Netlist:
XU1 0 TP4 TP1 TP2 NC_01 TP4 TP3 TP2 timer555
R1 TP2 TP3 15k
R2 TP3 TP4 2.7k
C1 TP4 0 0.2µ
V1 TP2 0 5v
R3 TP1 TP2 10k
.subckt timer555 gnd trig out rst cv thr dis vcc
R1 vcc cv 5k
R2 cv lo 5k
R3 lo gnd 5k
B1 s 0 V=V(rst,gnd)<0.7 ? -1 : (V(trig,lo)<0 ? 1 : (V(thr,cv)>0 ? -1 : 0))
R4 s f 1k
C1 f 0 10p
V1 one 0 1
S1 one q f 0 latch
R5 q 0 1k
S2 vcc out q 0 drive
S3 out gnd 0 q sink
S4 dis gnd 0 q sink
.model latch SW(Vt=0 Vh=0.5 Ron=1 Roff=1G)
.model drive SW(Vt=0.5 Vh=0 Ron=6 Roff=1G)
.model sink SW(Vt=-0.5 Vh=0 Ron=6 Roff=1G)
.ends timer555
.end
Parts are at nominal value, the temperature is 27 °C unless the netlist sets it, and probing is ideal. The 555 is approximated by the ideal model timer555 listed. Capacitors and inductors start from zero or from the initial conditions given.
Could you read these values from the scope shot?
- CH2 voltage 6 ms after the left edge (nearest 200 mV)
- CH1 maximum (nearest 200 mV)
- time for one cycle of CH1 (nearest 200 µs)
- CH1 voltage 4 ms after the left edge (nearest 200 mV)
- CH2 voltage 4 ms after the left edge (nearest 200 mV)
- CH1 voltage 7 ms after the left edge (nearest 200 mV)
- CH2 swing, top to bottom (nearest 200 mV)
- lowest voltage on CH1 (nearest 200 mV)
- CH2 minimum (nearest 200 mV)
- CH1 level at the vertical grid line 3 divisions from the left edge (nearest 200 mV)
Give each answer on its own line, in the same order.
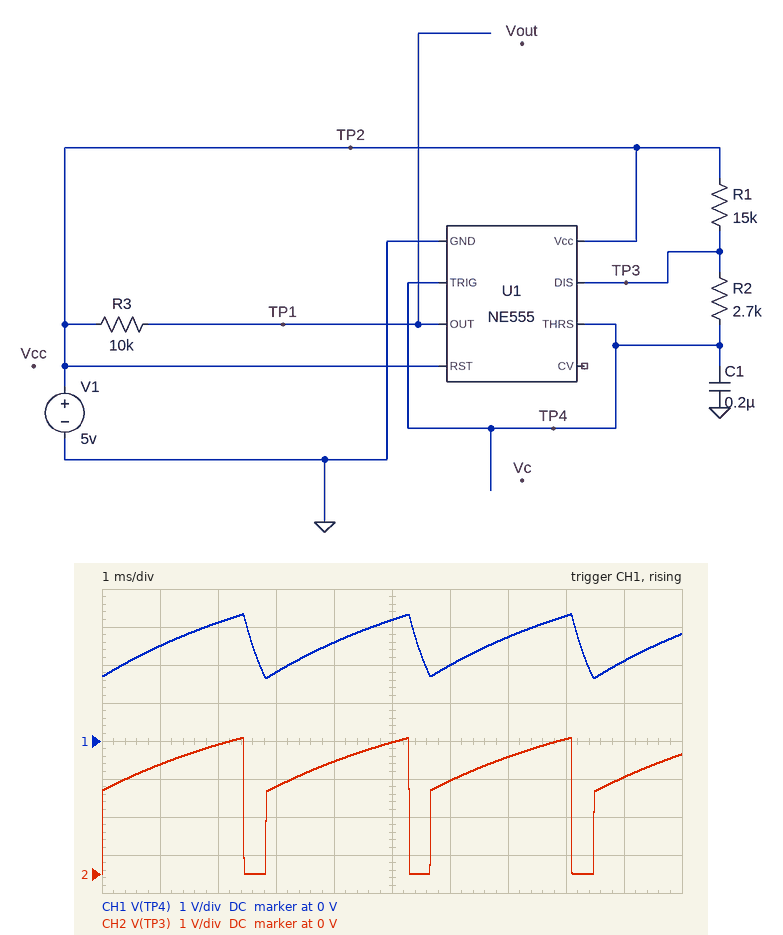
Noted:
2.4 V
3.4 V
2.8 ms
2.6 V
3.0 V
2.8 V
3.6 V
1.6 V
0 V
1.8 V
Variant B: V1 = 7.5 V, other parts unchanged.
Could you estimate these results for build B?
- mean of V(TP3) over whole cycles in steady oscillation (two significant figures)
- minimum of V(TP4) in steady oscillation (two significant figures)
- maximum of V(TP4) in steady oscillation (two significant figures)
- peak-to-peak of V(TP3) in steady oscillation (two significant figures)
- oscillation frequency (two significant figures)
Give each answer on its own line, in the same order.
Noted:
3.9 V
2.5 V
5.0 V
5.4 V
350 Hz
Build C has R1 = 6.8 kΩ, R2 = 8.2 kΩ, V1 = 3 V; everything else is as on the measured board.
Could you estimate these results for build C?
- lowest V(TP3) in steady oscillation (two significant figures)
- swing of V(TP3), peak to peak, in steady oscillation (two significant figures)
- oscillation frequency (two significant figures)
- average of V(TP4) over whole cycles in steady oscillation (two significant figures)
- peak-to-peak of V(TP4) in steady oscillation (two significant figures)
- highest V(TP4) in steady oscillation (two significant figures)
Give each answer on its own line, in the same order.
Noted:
3.4 mV
2.5 V
310 Hz
1.5 V
1.0 V
2.0 V
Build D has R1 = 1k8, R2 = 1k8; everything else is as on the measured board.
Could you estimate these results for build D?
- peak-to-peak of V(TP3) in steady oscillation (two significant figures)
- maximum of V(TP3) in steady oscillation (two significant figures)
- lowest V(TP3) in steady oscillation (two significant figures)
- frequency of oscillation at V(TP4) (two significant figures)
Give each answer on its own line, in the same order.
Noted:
4.1 V
4.2 V
22 mV
1.3 kHz
